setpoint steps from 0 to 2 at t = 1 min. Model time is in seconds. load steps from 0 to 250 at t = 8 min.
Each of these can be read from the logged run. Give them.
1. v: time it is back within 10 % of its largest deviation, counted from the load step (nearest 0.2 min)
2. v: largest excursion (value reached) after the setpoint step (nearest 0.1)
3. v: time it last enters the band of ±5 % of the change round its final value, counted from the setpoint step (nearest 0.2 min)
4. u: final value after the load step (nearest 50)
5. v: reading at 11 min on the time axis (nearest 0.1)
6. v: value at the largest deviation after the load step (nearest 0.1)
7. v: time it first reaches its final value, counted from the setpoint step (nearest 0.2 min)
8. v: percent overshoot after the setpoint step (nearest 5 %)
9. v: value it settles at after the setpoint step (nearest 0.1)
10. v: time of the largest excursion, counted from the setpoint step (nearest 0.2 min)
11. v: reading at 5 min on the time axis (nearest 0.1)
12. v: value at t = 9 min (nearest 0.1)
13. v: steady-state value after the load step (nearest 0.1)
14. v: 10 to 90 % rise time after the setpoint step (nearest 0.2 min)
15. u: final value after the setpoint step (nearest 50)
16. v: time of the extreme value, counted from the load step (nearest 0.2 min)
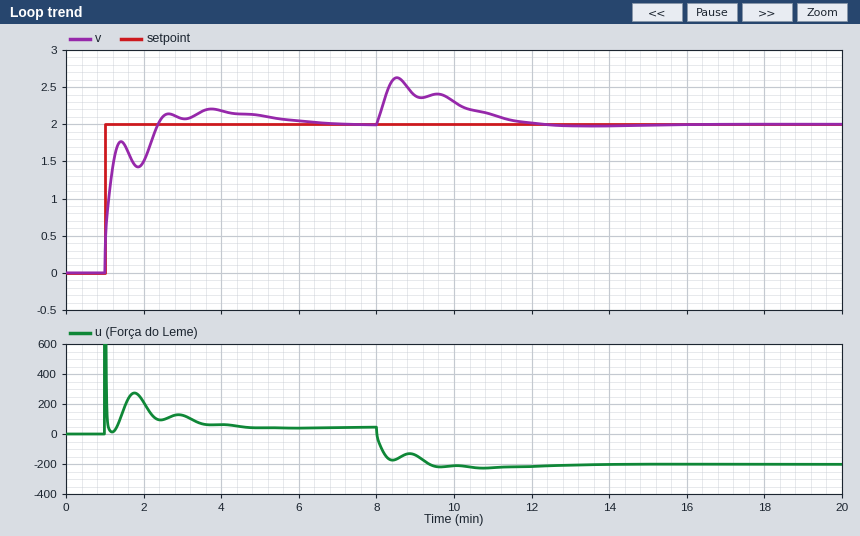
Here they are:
3.4 min
2.2
4.2 min
-200
2.1
2.6
1.4 min
10 %
2.0
2.8 min
2.1
2.4
2.0
1.2 min
50
0.6 min
